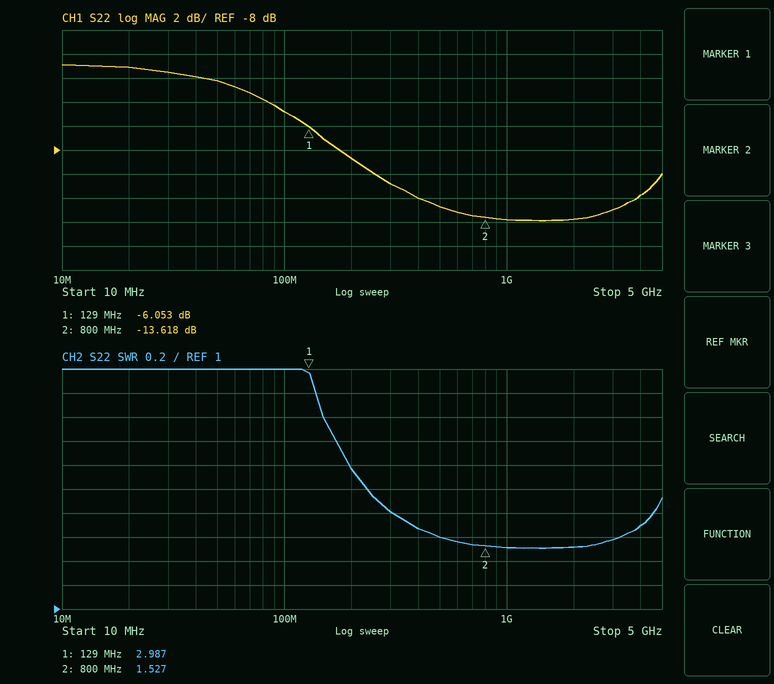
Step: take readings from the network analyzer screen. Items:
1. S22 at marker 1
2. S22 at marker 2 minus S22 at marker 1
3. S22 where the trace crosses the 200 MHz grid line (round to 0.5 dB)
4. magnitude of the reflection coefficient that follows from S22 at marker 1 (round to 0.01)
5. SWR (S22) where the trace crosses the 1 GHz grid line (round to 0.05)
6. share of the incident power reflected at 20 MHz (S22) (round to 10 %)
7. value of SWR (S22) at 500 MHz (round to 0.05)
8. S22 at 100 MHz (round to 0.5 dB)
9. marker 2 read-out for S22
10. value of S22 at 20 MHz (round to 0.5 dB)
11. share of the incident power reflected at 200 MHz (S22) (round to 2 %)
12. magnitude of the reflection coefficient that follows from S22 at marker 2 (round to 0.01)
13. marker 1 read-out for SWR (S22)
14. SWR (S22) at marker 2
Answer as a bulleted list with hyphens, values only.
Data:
- -6.053 dB
- -7.565 dB
- -8.5 dB
- 0.50
- 1.50
- 80 %
- 1.60
- -5.0 dB
- -13.618 dB
- -1.0 dB
- 14 %
- 0.21
- 2.987
- 1.527
